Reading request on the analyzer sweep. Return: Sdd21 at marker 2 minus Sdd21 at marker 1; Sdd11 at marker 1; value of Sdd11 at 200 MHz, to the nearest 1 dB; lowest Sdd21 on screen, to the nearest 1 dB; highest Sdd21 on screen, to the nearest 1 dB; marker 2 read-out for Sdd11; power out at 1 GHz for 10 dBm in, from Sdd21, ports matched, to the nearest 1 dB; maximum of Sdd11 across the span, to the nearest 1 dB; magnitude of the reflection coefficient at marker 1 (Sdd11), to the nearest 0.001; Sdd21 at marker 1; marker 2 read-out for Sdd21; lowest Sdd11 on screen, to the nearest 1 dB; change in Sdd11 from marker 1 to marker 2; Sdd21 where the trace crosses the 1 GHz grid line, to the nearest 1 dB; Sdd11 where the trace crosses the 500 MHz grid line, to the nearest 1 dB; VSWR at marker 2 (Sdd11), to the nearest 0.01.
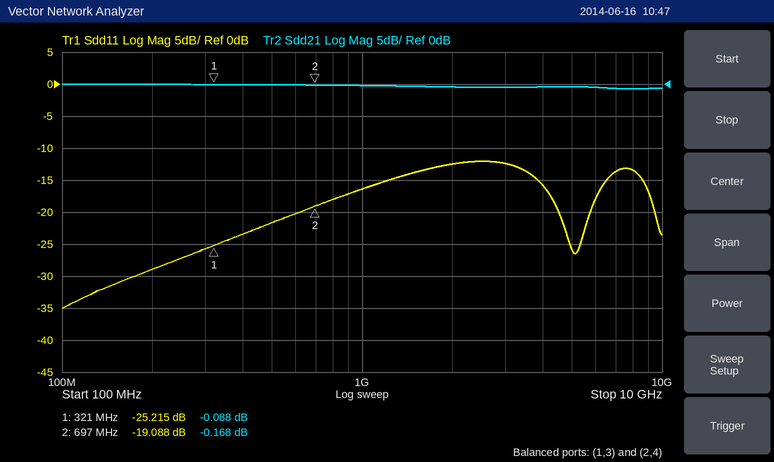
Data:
-0.080 dB
-25.215 dB
-29 dB
-1 dB
0 dB
-19.088 dB
10 dBm
-12 dB
0.055
-0.088 dB
-0.168 dB
-35 dB
6.127 dB
0 dB
-22 dB
1.25
